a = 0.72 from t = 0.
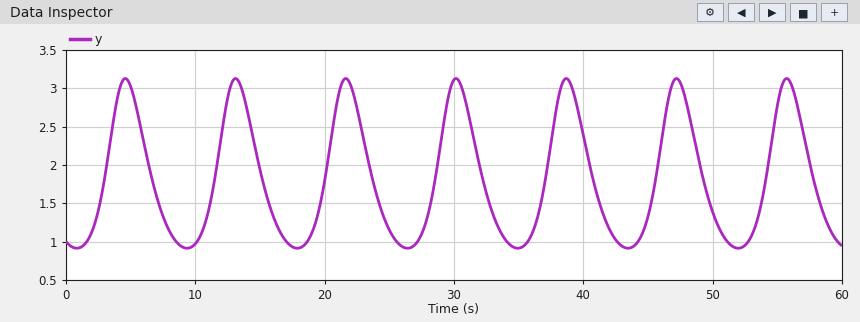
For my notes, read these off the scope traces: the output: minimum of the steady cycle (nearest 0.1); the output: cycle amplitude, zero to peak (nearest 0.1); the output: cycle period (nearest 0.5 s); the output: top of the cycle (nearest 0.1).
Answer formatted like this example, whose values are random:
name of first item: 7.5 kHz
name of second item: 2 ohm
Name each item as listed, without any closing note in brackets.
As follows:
the output: minimum of the steady cycle: 0.9
the output: cycle amplitude, zero to peak: 1.1
the output: cycle period: 8.5 s
the output: top of the cycle: 3.1
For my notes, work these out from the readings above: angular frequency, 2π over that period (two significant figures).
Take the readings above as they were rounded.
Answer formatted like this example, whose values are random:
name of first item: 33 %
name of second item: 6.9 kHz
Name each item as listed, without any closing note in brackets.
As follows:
angular frequency, 2π over that period: 0.74 rad/s
